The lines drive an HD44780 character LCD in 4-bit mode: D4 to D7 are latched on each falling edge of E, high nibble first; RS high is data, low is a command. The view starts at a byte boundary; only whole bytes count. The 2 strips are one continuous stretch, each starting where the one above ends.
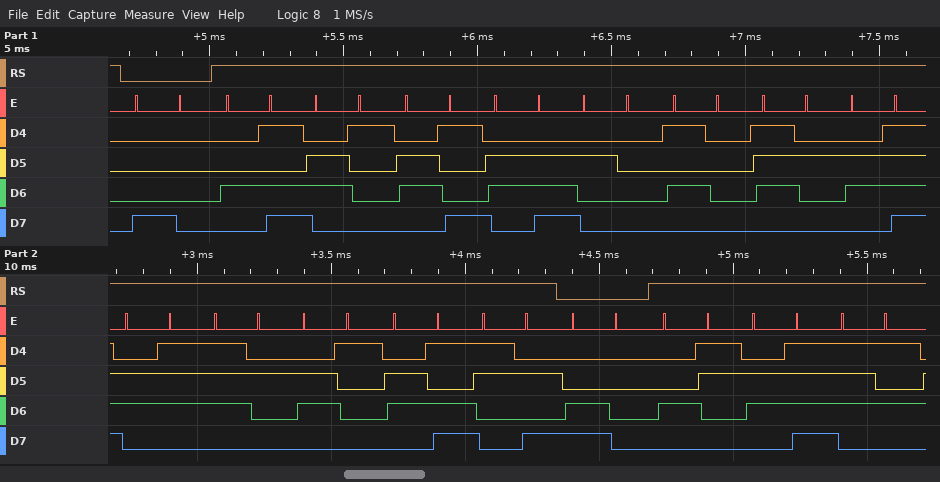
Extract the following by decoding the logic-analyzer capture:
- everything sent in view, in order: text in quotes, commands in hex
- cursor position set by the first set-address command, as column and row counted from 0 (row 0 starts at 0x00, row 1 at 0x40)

0x80 "Main Program:" 0xC0 "Cou"
column 0, row 0
